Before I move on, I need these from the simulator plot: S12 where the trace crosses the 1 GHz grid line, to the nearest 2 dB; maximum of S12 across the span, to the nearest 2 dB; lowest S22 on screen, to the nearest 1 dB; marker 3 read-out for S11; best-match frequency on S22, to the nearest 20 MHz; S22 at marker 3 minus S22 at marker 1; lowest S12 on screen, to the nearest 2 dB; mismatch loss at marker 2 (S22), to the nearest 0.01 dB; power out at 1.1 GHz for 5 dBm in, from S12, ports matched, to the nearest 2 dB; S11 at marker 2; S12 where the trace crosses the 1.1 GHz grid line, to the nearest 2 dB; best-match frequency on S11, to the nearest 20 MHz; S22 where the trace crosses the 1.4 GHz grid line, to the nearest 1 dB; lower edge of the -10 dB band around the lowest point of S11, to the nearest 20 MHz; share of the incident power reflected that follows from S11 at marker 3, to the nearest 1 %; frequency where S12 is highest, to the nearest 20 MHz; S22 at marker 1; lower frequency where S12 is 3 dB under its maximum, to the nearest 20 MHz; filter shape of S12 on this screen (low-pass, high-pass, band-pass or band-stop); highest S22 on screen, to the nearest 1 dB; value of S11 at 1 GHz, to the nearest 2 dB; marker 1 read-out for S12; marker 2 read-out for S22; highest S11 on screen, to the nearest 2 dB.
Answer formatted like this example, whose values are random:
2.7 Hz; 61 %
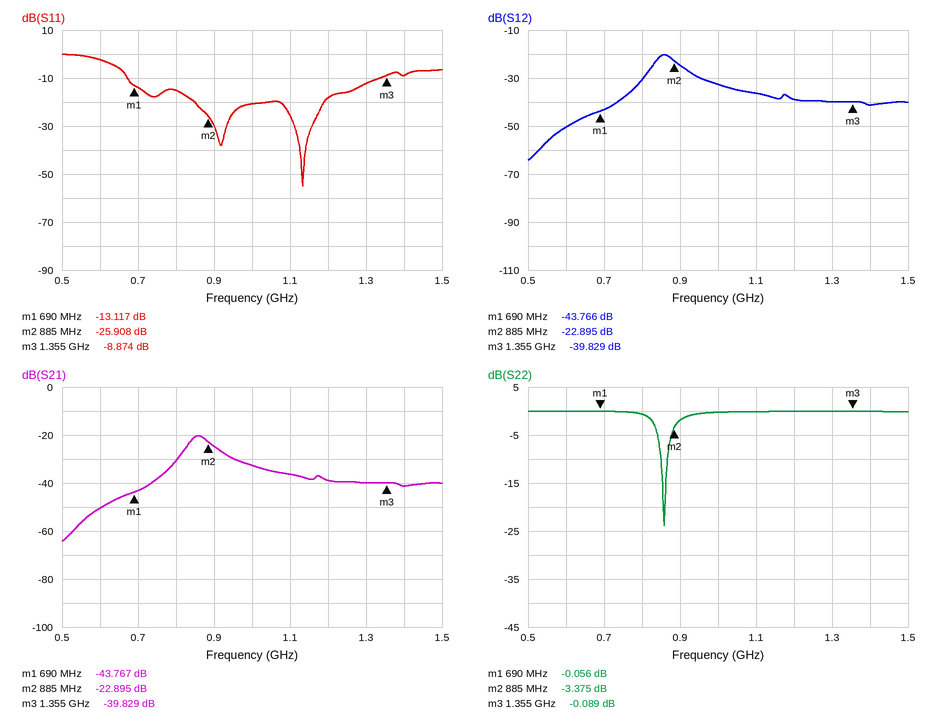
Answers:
-32 dB; -20 dB; -24 dB; -8.874 dB; 860 MHz; -0.033 dB; -64 dB; 2.67 dB; -32 dBm; -25.908 dB; -36 dB; 1.14 GHz; 0 dB; 680 MHz; 13 %; 860 MHz; -0.056 dB; 840 MHz; band-pass; 0 dB; -20 dB; -43.766 dB; -3.375 dB; 0 dB
